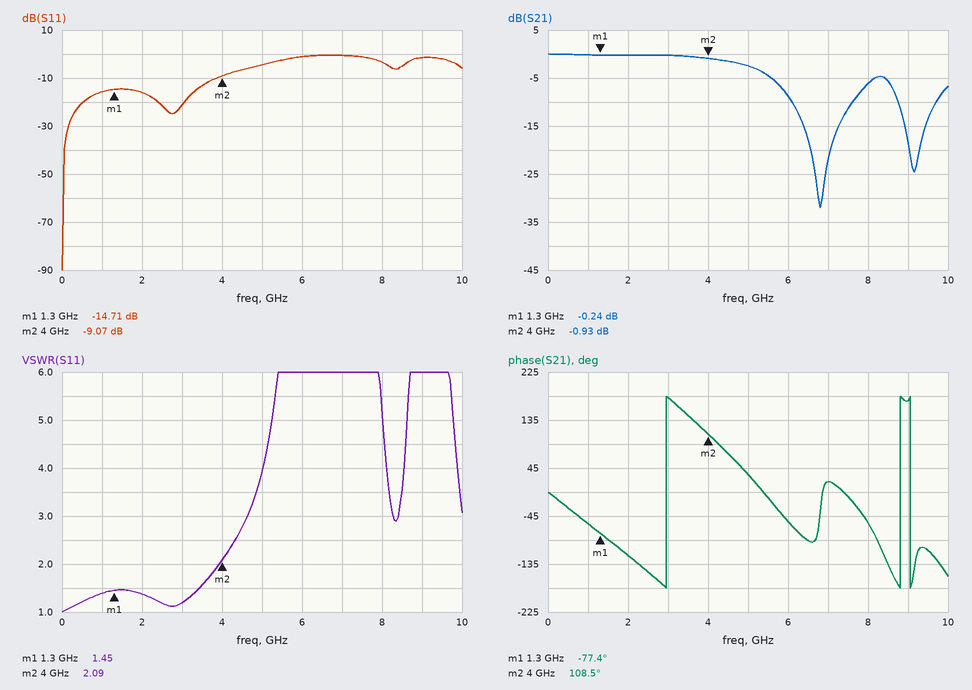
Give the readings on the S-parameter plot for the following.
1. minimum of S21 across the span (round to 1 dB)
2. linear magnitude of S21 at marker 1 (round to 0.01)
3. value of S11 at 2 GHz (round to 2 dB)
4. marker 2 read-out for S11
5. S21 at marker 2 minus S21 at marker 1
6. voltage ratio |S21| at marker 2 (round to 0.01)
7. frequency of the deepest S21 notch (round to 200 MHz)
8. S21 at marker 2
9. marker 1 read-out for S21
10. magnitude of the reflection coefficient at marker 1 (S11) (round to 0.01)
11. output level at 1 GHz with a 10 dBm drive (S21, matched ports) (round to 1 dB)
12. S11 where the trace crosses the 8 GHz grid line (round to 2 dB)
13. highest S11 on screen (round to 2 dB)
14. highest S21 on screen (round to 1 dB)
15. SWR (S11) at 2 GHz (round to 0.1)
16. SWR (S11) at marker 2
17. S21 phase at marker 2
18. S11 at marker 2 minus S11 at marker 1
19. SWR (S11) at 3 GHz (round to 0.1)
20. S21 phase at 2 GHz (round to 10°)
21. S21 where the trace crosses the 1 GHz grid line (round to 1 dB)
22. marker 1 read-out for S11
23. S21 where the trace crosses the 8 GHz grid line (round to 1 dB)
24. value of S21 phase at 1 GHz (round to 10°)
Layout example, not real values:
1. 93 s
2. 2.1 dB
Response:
1. -32 dB
2. 0.97
3. -16 dB
4. -9.07 dB
5. -0.69 dB
6. 0.90
7. 6.8 GHz
8. -0.93 dB
9. -0.24 dB
10. 0.18
11. 10 dBm
12. -4 dB
13. 0 dB
14. 0 dB
15. 1.4
16. 2.09
17. 108.5°
18. 5.64 dB
19. 1.2
20. -120°
21. 0 dB
22. -14.71 dB
23. -6 dB
24. -60°
